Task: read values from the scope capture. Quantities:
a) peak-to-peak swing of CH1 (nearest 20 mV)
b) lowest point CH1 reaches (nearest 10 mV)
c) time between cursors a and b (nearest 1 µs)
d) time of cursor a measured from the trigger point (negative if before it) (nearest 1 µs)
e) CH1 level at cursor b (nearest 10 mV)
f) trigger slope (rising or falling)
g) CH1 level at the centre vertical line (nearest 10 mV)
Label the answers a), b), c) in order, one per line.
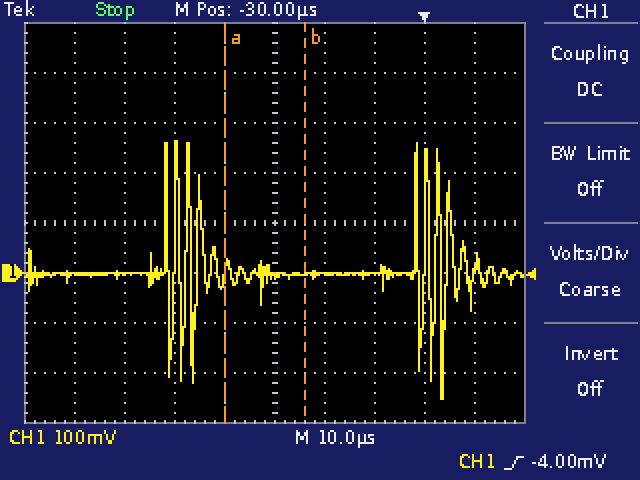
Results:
a) 520 mV
b) -250 mV
c) 16 µs
d) -40 µs
e) 0 mV
f) rising
g) -10 mV
